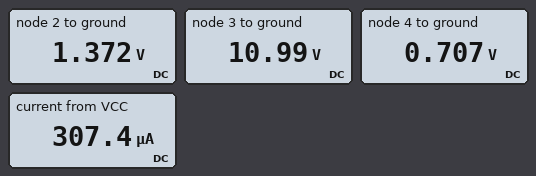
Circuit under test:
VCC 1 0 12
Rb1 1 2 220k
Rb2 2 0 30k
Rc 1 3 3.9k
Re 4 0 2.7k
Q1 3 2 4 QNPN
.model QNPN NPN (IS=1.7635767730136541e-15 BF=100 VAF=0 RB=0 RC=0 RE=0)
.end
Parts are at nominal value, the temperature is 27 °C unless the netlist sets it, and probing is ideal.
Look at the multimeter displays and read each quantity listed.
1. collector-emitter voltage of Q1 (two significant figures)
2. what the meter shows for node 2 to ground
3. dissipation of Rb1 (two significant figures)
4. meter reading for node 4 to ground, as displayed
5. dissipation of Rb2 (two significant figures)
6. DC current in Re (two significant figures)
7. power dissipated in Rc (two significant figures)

10 V
1.372 V
510 µW
0.707 V
63 µW
260 µA
260 µW
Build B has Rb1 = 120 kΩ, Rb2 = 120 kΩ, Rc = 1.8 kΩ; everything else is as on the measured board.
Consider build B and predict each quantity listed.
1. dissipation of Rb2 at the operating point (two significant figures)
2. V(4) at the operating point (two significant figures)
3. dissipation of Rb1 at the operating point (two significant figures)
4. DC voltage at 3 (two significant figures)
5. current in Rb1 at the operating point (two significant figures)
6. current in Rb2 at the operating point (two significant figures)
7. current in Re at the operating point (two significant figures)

210 µW
4.3 V
400 µW
9.1 V
58 µA
42 µA
1.6 mA
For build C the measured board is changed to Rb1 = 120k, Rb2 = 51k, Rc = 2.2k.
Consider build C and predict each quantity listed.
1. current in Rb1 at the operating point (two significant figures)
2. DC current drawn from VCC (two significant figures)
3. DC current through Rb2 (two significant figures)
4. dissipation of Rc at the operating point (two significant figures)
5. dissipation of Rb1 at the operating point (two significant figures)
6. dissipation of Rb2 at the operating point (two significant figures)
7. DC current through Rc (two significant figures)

73 µA
1.0 mA
64 µA
1.9 mW
640 µW
210 µW
930 µA
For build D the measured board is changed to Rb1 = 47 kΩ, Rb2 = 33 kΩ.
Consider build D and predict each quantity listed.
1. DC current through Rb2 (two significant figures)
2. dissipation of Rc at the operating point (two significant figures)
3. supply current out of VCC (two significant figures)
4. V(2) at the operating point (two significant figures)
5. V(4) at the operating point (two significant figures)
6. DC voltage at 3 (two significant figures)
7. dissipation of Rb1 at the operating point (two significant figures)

140 µA
8.2 mW
1.6 mA
4.7 V
4.0 V
6.3 V
1.1 mW
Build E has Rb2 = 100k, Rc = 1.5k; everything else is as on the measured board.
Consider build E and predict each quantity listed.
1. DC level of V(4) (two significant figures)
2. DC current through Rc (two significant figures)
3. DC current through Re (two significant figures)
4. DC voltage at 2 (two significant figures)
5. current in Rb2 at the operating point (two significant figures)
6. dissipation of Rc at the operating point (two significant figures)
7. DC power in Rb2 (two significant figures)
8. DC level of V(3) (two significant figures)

2.4 V
890 µA
900 µA
3.1 V
31 µA
1.2 mW
98 µW
11 V
